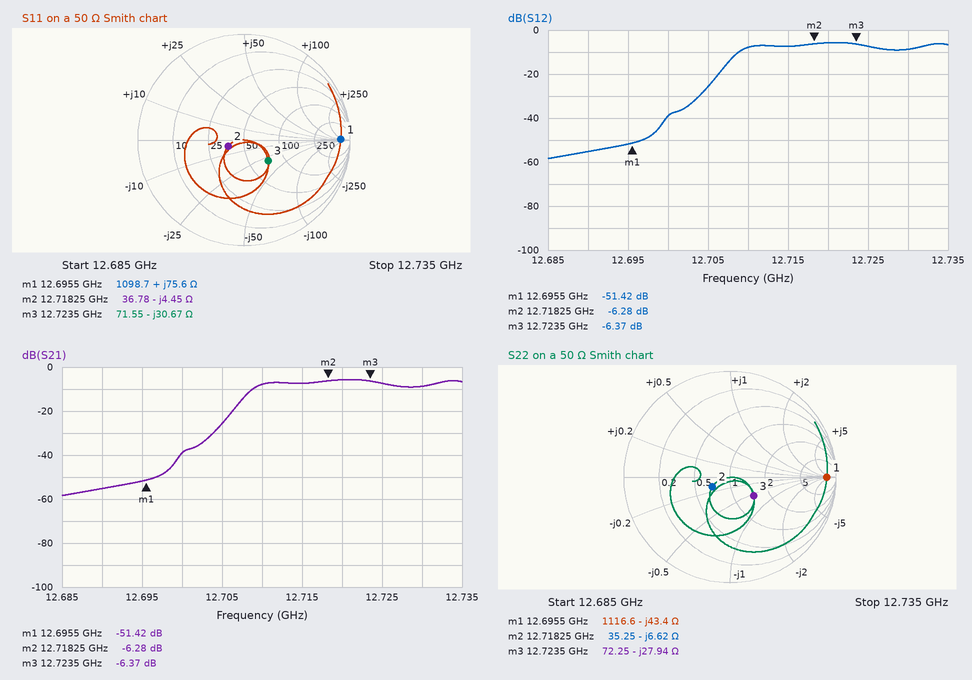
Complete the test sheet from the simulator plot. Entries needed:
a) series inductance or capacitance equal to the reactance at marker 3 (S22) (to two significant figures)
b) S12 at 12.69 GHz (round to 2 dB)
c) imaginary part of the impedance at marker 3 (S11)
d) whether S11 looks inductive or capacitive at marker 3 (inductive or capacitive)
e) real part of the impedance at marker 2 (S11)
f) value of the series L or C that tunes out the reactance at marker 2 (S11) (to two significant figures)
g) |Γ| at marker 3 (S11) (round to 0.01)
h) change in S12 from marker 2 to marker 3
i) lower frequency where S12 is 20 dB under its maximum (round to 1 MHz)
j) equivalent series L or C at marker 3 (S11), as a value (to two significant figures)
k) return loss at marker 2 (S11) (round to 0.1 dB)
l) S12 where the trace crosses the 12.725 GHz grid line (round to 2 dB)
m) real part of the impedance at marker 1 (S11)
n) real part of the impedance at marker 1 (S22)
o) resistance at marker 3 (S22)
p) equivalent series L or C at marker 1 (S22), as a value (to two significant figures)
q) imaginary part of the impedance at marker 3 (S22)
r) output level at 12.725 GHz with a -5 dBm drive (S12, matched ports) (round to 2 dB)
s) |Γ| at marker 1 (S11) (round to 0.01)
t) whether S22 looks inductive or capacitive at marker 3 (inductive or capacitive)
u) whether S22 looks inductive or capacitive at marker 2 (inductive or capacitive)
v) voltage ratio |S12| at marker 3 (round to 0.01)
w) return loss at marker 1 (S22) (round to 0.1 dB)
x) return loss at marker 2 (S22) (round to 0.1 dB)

450 fF
-56 dB
-30.67 Ω
capacitive
36.78 Ω
56 pH
0.30
-0.09 dB
12.705 GHz
410 fF
15.9 dB
-8 dB
1098.7 Ω
1116.6 Ω
72.25 Ω
290 fF
-27.94 Ω
-12 dBm
0.91
capacitive
capacitive
0.48
0.8 dB
14.5 dB
